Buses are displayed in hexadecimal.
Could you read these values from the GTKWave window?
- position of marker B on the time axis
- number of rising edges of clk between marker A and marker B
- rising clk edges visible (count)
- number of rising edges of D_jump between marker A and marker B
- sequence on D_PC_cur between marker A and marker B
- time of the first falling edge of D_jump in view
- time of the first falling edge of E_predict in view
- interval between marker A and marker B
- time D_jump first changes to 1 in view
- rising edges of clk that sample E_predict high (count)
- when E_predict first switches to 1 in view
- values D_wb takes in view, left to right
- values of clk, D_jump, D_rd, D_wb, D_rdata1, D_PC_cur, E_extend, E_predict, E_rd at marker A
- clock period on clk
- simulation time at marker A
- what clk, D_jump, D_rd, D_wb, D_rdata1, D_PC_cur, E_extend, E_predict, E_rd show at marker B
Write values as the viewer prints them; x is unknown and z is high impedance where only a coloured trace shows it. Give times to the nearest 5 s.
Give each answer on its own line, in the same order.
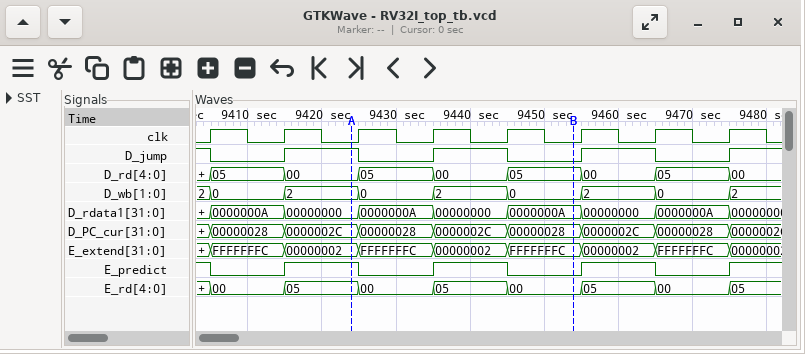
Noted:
9455 s
3
8
1
0000002C, 00000028, 0000002C, 00000028
9405 s
9405 s
30 s
9415 s
4
9415 s
2, 0, 2, 0, 2, 0, 2, 0, 2
clk=0, D_jump=1, D_rd=00, D_wb=2, D_rdata1=00000000, D_PC_cur=0000002C, E_extend=00000002, E_predict=1, E_rd=05
10 s
9425 s
clk=0, D_jump=0, D_rd=05, D_wb=0, D_rdata1=0000000A, D_PC_cur=00000028, E_extend=FFFFFFFC, E_predict=0, E_rd=00
